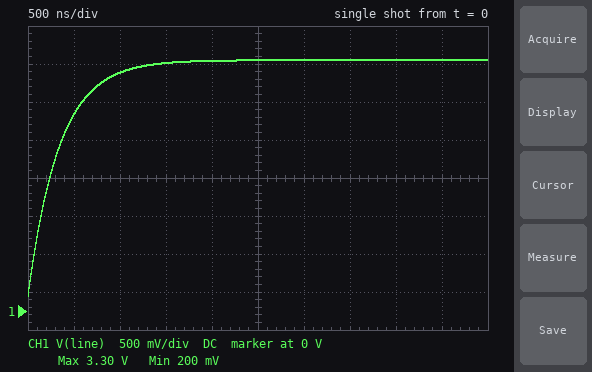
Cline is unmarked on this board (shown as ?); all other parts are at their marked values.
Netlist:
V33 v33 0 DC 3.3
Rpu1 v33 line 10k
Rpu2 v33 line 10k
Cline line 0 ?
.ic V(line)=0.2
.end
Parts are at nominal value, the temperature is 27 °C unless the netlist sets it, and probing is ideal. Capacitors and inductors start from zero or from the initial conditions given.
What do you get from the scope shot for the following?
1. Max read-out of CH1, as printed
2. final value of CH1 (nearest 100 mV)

3.30 V
3.3 V
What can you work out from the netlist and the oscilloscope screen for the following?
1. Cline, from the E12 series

68 pF
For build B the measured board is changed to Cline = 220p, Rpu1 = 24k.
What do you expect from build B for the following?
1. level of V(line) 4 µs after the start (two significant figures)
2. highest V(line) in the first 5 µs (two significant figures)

3.1 V
3.2 V
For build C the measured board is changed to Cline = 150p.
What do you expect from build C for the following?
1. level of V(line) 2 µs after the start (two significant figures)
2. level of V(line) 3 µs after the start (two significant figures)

3.1 V
3.2 V
